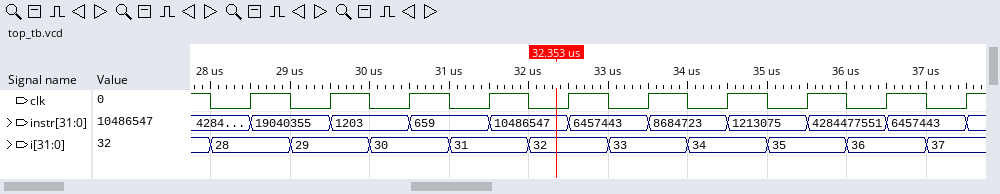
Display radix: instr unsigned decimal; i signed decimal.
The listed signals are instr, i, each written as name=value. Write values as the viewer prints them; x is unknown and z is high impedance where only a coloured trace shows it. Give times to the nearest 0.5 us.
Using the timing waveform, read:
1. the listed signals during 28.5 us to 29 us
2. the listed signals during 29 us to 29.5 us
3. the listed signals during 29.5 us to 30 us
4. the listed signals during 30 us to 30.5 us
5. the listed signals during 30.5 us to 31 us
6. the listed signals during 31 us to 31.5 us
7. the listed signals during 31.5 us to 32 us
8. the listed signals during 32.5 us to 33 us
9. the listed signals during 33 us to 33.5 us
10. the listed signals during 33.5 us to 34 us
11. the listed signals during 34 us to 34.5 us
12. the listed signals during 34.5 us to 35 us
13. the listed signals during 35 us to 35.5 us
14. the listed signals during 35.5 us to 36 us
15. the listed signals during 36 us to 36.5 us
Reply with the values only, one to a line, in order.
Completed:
instr=19040355, i=28
instr=19040355, i=29
instr=1203, i=29
instr=1203, i=30
instr=659, i=30
instr=659, i=31
instr=10486547, i=31
instr=6457443, i=32
instr=6457443, i=33
instr=8684723, i=33
instr=8684723, i=34
instr=1213075, i=34
instr=1213075, i=35
instr=4284477551, i=35
instr=4284477551, i=36
